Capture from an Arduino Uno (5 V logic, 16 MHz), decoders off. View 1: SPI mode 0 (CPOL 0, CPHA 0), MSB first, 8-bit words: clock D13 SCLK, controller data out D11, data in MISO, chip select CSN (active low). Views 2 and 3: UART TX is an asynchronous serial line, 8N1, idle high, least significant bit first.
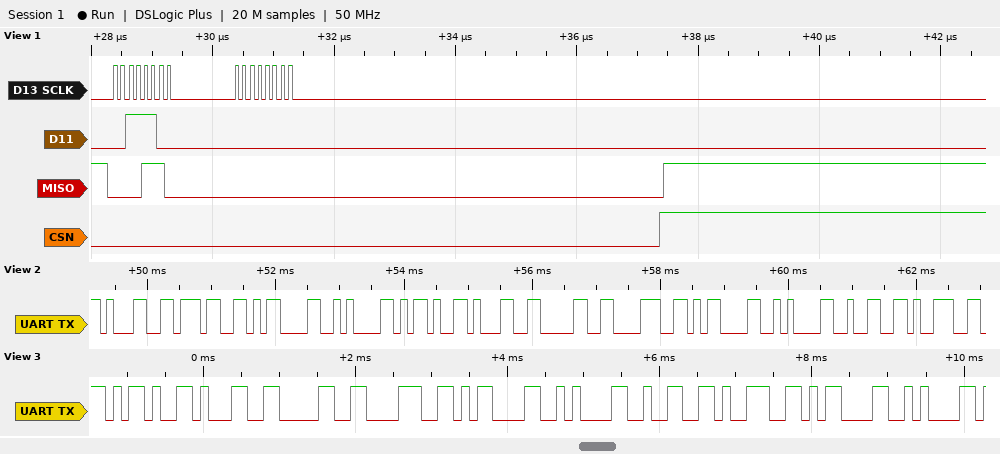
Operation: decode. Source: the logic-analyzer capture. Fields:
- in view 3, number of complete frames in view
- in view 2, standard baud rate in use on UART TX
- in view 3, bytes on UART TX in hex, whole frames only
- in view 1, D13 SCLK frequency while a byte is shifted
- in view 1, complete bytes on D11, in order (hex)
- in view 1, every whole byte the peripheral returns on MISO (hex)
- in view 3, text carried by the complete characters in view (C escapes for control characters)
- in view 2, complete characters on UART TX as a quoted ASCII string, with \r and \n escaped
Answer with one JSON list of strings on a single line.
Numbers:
["10", "9600 baud", "0x2D 0x31 0x30 0x38 0x0D 0x0A 0x32 0x39 0x0D 0x0A", "8 MHz", "3C 00", "0E 00", "\"-108\\r\\n29\\r\\n\"", "\"17\\r\\n-108\\r\\n29\""]
